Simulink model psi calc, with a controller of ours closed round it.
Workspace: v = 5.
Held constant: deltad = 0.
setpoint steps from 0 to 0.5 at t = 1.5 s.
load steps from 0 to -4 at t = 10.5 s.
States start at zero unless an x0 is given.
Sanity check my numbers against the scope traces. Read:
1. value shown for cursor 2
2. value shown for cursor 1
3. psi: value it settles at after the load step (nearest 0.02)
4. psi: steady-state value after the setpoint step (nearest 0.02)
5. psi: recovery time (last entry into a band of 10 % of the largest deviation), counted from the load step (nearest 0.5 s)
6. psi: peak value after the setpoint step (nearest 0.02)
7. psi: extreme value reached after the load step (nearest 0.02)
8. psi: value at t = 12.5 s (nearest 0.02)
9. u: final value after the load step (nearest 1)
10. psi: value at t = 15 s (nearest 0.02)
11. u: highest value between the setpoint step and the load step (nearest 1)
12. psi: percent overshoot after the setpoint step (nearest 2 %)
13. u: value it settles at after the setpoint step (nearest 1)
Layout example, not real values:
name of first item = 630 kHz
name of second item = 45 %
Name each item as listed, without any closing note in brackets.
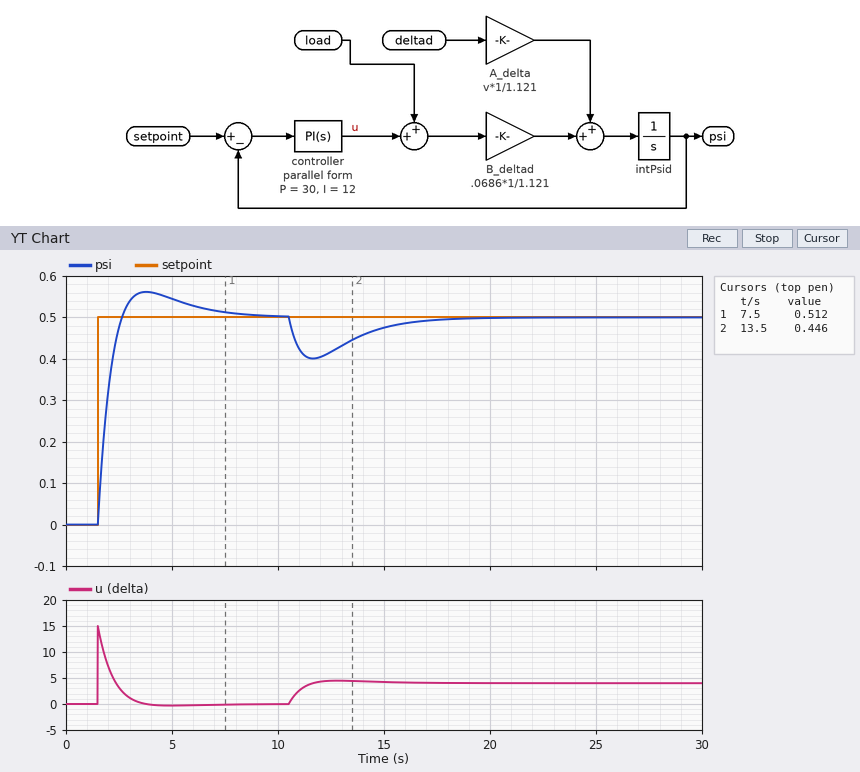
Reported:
value shown for cursor 2 = 0.446
value shown for cursor 1 = 0.512
psi: value it settles at after the load step = 0.50
psi: steady-state value after the setpoint step = 0.50
psi: recovery time (last entry into a band of 10 % of the largest deviation), counted from the load step = 6.0 s
psi: peak value after the setpoint step = 0.56
psi: extreme value reached after the load step = 0.40
psi: value at t = 12.5 s = 0.42
u: final value after the load step = 4
psi: value at t = 15 s = 0.48
u: highest value between the setpoint step and the load step = 15
psi: percent overshoot after the setpoint step = 12 %
u: value it settles at after the setpoint step = 0
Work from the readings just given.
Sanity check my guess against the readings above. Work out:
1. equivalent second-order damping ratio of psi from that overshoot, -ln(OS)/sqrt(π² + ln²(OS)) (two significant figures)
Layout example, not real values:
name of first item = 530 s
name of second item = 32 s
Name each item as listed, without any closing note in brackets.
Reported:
equivalent second-order damping ratio of psi from that overshoot, -ln(OS)/sqrt(π² + ln²(OS)) = 0.56
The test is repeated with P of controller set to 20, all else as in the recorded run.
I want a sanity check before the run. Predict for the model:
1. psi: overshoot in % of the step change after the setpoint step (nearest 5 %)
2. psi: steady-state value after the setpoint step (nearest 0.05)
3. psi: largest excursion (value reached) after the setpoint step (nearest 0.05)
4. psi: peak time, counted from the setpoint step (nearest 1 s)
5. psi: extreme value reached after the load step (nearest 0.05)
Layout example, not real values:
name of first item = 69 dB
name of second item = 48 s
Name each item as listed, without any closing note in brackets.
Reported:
psi: overshoot in % of the step change after the setpoint step = 20 %
psi: steady-state value after the setpoint step = 0.50
psi: largest excursion (value reached) after the setpoint step = 0.60
psi: peak time, counted from the setpoint step = 3 s
psi: extreme value reached after the load step = 0.35
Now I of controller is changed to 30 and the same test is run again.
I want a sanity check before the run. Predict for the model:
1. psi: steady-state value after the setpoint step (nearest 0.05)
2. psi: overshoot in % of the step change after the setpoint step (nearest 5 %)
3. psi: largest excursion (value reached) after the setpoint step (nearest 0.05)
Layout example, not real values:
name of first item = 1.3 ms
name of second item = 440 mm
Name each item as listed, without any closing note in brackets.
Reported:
psi: steady-state value after the setpoint step = 0.50
psi: overshoot in % of the step change after the setpoint step = 20 %
psi: largest excursion (value reached) after the setpoint step = 0.60
